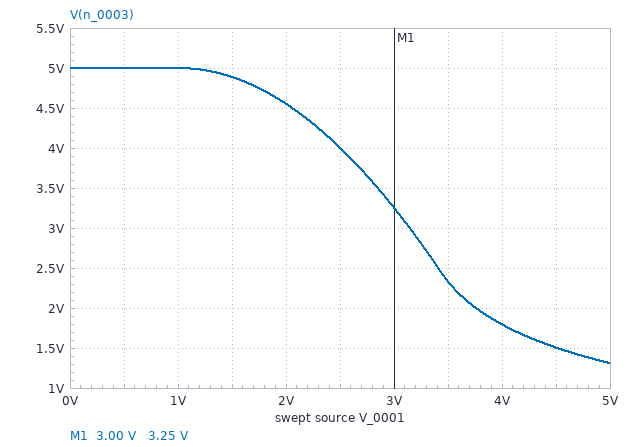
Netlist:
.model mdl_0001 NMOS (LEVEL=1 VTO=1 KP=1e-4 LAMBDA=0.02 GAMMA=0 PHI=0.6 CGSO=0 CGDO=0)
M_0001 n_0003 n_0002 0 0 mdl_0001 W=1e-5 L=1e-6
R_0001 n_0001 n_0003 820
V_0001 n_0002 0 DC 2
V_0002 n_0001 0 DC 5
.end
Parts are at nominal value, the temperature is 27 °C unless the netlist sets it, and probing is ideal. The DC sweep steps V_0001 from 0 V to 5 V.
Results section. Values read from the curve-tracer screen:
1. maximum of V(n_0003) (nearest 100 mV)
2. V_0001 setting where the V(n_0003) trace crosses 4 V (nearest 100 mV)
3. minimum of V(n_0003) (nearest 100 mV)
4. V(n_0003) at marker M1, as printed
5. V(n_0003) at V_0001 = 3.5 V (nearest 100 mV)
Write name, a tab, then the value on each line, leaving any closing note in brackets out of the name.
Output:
maximum of V(n_0003)	5.0 V
V_0001 setting where the V(n_0003) trace crosses 4 V	2.5 V
minimum of V(n_0003)	1.3 V
V(n_0003) at marker M1, as printed	3.25 V
V(n_0003) at V_0001 = 3.5 V	2.3 V
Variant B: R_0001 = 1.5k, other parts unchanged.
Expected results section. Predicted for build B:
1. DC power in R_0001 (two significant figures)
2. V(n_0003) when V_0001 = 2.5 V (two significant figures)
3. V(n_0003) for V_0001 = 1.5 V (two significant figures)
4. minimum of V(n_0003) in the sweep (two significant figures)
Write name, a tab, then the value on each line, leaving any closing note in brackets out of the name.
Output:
DC power in R_0001	440 µW
V(n_0003) when V_0001 = 2.5 V	3.2 V
V(n_0003) for V_0001 = 1.5 V	4.8 V
minimum of V(n_0003) in the sweep	770 mV
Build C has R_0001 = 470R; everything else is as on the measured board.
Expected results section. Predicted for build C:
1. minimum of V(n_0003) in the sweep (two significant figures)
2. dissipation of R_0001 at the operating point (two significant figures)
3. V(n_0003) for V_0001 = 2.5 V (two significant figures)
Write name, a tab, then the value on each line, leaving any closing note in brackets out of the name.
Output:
minimum of V(n_0003) in the sweep	2.0 V
dissipation of R_0001 at the operating point	140 µW
V(n_0003) for V_0001 = 2.5 V	4.4 V
